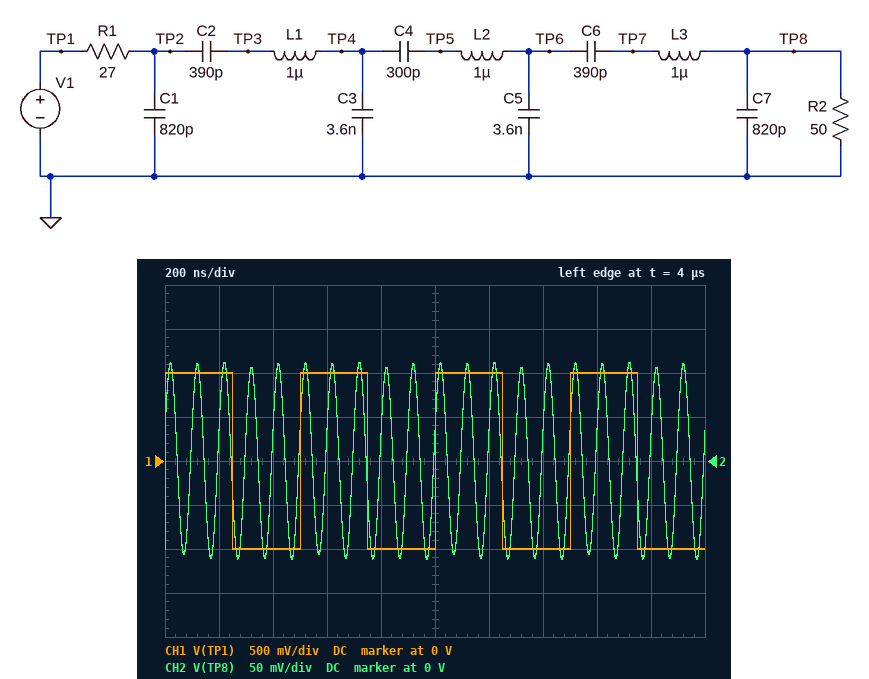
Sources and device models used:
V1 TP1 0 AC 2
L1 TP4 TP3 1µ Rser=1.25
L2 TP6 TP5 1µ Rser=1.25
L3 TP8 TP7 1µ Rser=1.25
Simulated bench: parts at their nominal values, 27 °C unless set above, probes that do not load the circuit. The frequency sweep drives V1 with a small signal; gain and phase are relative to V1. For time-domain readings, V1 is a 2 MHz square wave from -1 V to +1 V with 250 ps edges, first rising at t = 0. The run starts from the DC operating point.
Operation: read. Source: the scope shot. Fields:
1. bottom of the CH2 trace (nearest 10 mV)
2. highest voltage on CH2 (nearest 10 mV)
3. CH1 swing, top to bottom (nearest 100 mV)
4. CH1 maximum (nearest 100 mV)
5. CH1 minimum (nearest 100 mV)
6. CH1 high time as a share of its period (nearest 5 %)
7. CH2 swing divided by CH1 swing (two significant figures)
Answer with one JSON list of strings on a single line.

["-110 mV", "110 mV", "2.0 V", "1.0 V", "-1.0 V", "50 %", "0.11"]
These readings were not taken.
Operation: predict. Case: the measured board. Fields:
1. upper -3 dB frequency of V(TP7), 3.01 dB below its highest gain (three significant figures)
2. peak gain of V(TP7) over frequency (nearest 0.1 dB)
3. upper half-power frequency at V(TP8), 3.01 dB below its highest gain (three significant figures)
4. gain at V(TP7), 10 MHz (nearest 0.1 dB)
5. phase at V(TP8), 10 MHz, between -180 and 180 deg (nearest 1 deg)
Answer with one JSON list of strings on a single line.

["10.4 MHz", "1.0 dB", "10.3 MHz", "1.0 dB", "27 deg"]
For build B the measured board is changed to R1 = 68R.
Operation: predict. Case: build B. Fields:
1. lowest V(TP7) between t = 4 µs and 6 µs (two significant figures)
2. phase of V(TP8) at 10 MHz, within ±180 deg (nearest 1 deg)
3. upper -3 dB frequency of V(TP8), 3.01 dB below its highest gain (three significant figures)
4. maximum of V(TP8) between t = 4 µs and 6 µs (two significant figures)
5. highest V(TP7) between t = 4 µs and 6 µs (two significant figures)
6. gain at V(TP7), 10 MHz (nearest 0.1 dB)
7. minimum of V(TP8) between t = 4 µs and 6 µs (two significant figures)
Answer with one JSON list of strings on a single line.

["-190 mV", "28 deg", "10.4 MHz", "73 mV", "190 mV", "-2.7 dB", "-73 mV"]
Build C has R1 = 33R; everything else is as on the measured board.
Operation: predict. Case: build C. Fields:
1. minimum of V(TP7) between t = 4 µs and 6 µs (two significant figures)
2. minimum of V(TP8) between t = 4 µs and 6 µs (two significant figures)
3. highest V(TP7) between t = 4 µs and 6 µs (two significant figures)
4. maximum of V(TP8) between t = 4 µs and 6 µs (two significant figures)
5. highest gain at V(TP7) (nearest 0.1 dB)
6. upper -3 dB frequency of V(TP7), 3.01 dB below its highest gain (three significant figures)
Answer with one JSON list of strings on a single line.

["-270 mV", "-100 mV", "270 mV", "100 mV", "0.3 dB", "10.4 MHz"]
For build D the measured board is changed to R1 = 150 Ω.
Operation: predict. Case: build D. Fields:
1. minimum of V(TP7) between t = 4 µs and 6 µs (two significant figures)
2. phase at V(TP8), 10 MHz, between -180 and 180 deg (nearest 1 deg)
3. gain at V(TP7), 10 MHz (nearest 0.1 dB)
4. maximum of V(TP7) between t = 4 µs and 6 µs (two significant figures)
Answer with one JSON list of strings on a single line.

["-110 mV", "28 deg", "-7.3 dB", "110 mV"]
